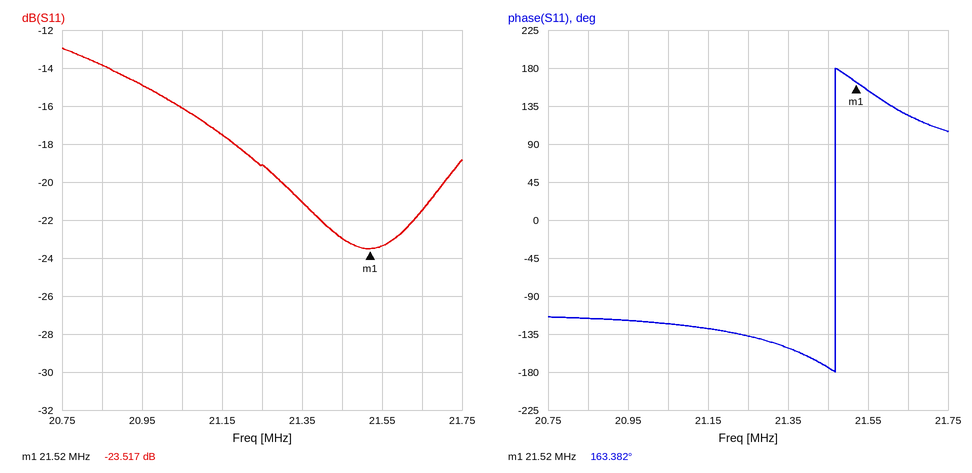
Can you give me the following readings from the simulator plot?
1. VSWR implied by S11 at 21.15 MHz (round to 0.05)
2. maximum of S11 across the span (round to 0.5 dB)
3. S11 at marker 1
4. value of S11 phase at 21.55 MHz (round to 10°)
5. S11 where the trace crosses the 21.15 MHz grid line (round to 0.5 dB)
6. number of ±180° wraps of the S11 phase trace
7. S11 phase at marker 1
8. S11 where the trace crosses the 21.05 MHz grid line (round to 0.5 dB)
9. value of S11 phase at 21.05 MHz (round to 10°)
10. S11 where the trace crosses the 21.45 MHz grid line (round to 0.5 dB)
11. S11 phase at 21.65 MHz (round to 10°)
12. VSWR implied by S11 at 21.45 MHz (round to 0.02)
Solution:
1.30
-13.0 dB
-23.517 dB
150°
-17.5 dB
1
163.382°
-16.0 dB
-120°
-23.0 dB
120°
1.16
